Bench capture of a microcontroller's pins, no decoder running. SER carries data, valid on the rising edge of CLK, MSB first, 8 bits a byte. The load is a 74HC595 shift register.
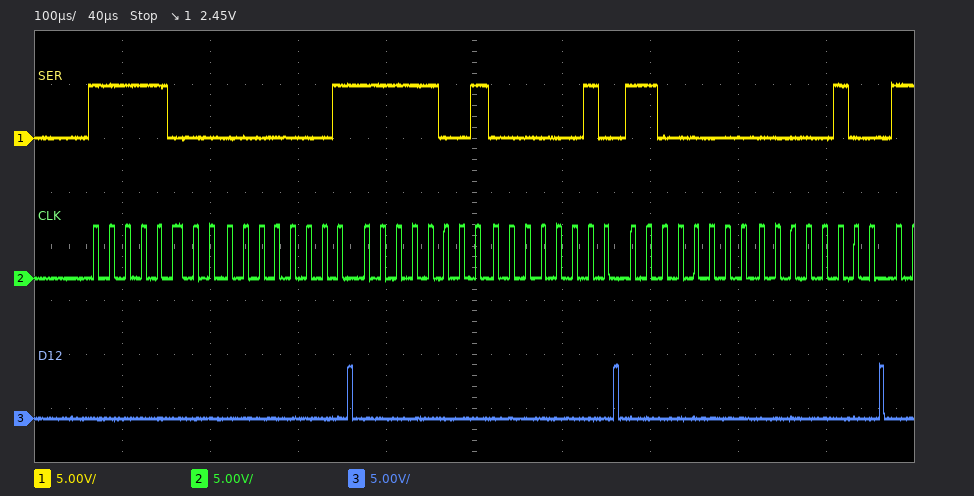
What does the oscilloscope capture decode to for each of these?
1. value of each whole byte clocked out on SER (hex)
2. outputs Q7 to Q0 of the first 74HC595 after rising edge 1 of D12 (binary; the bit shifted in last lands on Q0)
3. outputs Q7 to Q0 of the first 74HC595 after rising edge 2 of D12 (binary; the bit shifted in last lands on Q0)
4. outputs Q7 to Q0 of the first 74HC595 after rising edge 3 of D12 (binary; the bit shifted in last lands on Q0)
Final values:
F8 01 F9 02 C0 04
00000001
00000010
00000100
